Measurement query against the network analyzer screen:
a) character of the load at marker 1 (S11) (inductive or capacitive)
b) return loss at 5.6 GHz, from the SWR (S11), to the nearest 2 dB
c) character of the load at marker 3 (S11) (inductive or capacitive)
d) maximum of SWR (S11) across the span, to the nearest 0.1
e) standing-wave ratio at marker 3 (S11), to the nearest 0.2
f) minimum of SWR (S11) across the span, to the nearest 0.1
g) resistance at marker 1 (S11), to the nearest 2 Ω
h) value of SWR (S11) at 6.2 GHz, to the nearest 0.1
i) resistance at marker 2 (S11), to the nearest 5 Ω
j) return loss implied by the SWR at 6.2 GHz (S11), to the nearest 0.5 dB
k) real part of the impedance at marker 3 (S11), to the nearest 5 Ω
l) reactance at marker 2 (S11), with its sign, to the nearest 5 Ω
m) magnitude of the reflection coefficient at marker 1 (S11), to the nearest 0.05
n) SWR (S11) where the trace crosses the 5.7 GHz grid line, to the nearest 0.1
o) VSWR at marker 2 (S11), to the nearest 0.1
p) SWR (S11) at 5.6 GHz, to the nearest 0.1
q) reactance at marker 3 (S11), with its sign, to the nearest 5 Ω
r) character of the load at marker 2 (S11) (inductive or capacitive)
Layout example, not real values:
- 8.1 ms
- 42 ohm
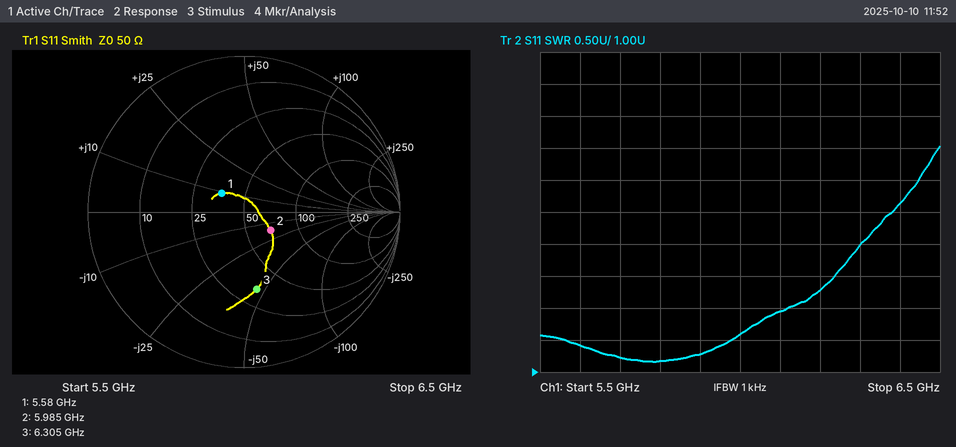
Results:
- inductive
- 16 dB
- capacitive
- 4.5
- 3.0
- 1.2
- 36 Ω
- 2.3
- 70 Ω
- 8.0 dB
- 35 Ω
- -15 Ω
- 0.20
- 1.2
- 1.5
- 1.4
- -45 Ω
- capacitive
